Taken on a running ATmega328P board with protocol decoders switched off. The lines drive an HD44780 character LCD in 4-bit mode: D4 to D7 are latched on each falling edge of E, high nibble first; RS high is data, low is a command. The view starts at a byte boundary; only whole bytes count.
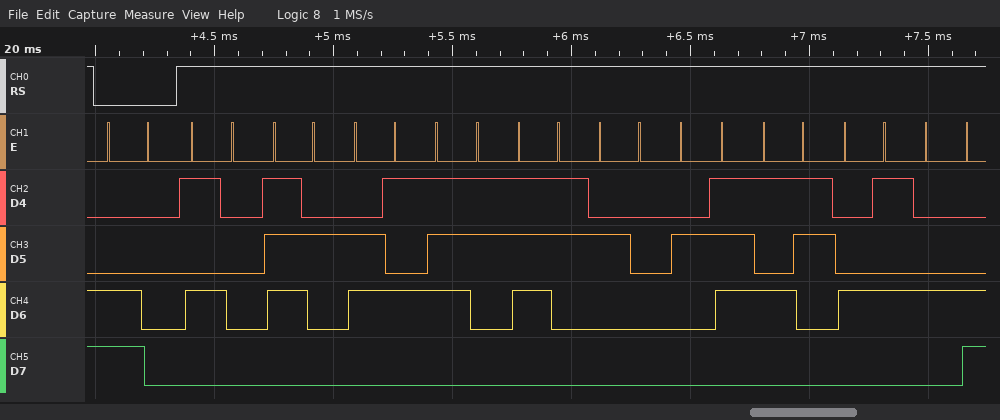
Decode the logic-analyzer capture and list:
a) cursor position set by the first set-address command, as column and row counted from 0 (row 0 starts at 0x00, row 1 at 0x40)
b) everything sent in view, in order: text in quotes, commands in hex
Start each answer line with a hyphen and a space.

- column 0, row 1
- 0xC0 "Press 'SEL"
